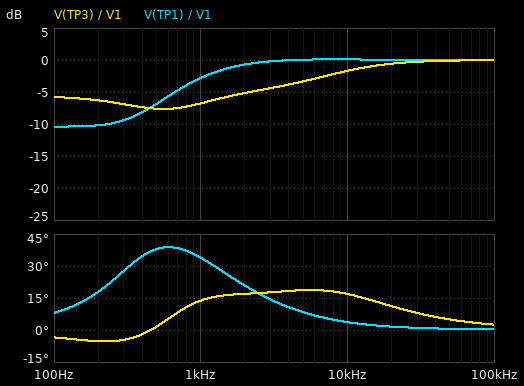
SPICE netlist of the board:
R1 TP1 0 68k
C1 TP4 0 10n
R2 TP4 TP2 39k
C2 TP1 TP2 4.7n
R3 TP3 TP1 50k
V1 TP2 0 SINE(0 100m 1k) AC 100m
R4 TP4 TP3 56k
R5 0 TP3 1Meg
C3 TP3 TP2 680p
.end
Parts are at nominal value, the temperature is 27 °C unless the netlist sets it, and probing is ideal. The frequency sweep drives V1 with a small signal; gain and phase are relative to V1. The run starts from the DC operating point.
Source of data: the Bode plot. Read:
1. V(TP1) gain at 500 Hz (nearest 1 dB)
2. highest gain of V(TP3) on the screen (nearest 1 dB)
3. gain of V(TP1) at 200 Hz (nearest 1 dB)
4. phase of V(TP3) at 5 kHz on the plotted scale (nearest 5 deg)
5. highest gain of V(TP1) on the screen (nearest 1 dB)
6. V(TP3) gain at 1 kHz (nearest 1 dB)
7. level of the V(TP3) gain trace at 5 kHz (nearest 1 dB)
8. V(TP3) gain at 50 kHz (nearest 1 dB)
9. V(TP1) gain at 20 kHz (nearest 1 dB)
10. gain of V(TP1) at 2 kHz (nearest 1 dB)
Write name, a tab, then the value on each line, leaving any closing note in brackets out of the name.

V(TP1) gain at 500 Hz	-7 dB
highest gain of V(TP3) on the screen	0 dB
gain of V(TP1) at 200 Hz	-10 dB
phase of V(TP3) at 5 kHz on the plotted scale	20 deg
highest gain of V(TP1) on the screen	0 dB
V(TP3) gain at 1 kHz	-7 dB
level of the V(TP3) gain trace at 5 kHz	-3 dB
V(TP3) gain at 50 kHz	0 dB
V(TP1) gain at 20 kHz	0 dB
gain of V(TP1) at 2 kHz	-1 dB
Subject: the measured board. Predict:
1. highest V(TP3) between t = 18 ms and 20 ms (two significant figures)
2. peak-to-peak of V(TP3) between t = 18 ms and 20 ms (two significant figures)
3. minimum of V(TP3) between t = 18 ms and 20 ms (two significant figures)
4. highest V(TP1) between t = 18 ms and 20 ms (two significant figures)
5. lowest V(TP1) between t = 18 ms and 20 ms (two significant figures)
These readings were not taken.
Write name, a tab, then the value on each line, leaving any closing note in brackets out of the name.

highest V(TP3) between t = 18 ms and 20 ms	46 mV
peak-to-peak of V(TP3) between t = 18 ms and 20 ms	92 mV
minimum of V(TP3) between t = 18 ms and 20 ms	-46 mV
highest V(TP1) between t = 18 ms and 20 ms	72 mV
lowest V(TP1) between t = 18 ms and 20 ms	-72 mV
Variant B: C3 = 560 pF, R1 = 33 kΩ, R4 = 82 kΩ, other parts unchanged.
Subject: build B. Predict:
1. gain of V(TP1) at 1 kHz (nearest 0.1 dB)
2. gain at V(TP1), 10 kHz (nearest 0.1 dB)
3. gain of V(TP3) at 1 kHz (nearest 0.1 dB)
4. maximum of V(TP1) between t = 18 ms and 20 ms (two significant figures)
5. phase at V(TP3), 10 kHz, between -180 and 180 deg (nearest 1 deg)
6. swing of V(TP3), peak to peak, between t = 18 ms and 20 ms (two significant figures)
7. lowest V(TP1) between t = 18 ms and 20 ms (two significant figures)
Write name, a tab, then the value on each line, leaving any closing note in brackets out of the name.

gain of V(TP1) at 1 kHz	-4.6 dB
gain at V(TP1), 10 kHz	0 dB
gain of V(TP3) at 1 kHz	-7.8 dB
maximum of V(TP1) between t = 18 ms and 20 ms	59 mV
phase at V(TP3), 10 kHz, between -180 and 180 deg	15 deg
swing of V(TP3), peak to peak, between t = 18 ms and 20 ms	82 mV
lowest V(TP1) between t = 18 ms and 20 ms	-59 mV
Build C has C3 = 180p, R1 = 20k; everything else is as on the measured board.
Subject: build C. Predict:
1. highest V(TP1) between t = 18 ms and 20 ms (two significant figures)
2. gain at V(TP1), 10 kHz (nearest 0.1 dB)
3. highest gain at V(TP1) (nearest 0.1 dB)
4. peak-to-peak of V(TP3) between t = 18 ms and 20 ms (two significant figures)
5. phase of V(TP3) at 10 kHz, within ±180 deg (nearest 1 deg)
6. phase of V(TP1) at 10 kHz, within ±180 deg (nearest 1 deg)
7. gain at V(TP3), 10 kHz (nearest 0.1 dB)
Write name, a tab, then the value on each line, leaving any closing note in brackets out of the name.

highest V(TP1) between t = 18 ms and 20 ms	41 mV
gain at V(TP1), 10 kHz	-0.1 dB
highest gain at V(TP1)	0 dB
peak-to-peak of V(TP3) between t = 18 ms and 20 ms	45 mV
phase of V(TP3) at 10 kHz, within ±180 deg	20 deg
phase of V(TP1) at 10 kHz, within ±180 deg	11 deg
gain at V(TP3), 10 kHz	-4.5 dB
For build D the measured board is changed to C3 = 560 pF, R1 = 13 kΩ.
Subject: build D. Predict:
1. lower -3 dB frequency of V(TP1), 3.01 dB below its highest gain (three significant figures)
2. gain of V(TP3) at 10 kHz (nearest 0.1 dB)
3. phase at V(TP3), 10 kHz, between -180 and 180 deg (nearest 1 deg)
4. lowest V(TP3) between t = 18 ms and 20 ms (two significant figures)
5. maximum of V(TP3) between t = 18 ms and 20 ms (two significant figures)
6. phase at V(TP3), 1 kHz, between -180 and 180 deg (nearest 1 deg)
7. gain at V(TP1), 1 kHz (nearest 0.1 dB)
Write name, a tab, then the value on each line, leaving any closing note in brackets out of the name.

lower -3 dB frequency of V(TP1), 3.01 dB below its highest gain	2.82 kHz
gain of V(TP3) at 10 kHz	-1.6 dB
phase at V(TP3), 10 kHz, between -180 and 180 deg	22 deg
lowest V(TP3) between t = 18 ms and 20 ms	-20 mV
maximum of V(TP3) between t = 18 ms and 20 ms	20 mV
phase at V(TP3), 1 kHz, between -180 and 180 deg	25 deg
gain at V(TP1), 1 kHz	-10.2 dB
